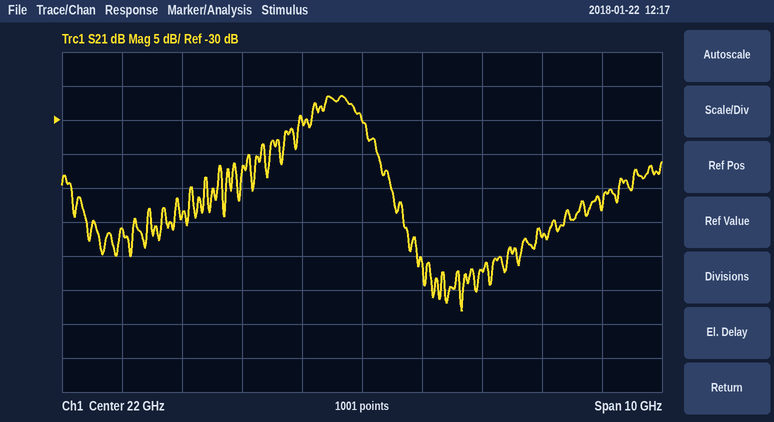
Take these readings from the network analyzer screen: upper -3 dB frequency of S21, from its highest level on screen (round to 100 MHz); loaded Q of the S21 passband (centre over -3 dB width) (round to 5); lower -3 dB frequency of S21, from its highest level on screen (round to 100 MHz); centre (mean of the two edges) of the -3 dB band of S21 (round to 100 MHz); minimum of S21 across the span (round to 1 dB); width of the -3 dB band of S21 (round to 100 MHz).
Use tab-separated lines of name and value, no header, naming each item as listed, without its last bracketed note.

upper -3 dB frequency of S21, from its highest level on screen	22.0 GHz
loaded Q of the S21 passband (centre over -3 dB width)	25
lower -3 dB frequency of S21, from its highest level on screen	21.2 GHz
centre (mean of the two edges) of the -3 dB band of S21	21.6 GHz
minimum of S21 across the span	-58 dB
width of the -3 dB band of S21	800 MHz
